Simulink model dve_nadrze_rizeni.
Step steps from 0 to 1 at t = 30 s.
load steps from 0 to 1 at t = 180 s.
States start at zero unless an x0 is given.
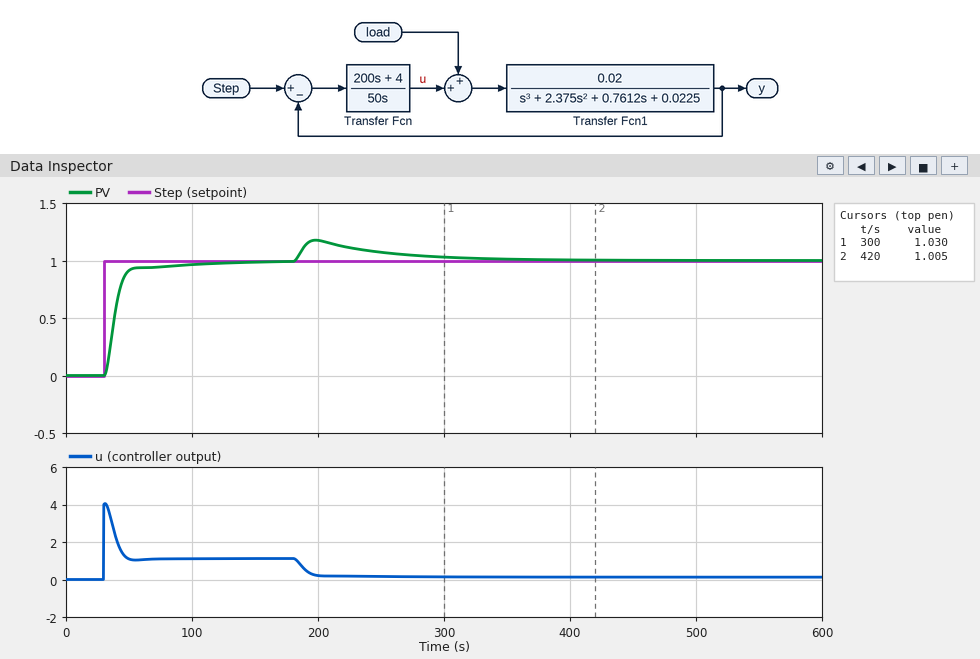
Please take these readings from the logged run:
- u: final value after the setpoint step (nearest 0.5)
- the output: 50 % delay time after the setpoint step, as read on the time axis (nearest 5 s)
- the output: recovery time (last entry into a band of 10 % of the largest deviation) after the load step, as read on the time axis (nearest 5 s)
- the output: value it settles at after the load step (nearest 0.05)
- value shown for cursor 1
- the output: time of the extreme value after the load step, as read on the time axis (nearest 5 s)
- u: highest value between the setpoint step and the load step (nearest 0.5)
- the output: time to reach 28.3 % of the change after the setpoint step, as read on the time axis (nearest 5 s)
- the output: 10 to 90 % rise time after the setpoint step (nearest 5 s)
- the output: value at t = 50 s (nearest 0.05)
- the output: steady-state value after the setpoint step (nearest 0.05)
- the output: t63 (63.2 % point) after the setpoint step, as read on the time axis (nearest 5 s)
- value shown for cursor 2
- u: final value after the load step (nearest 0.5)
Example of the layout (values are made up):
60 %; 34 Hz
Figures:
1.0; 40 s; 325 s; 1.00; 1.030; 200 s; 4.0; 35 s; 15 s; 0.90; 1.00; 40 s; 1.005; 0.0
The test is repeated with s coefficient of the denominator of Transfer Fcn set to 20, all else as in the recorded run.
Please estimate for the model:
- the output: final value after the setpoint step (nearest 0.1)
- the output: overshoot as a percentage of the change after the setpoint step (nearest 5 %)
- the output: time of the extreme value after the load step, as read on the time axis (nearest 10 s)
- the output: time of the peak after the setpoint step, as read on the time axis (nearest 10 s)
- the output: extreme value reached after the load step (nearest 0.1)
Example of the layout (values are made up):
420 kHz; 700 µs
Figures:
1.0; 15 %; 190 s; 40 s; 1.1
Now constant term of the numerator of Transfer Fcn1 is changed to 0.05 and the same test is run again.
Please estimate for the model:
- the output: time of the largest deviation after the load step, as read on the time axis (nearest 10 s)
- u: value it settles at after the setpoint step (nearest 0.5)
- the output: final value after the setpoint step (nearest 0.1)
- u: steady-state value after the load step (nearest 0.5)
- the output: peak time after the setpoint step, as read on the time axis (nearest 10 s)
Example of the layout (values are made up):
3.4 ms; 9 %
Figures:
190 s; 0.5; 1.0; -0.5; 40 s
